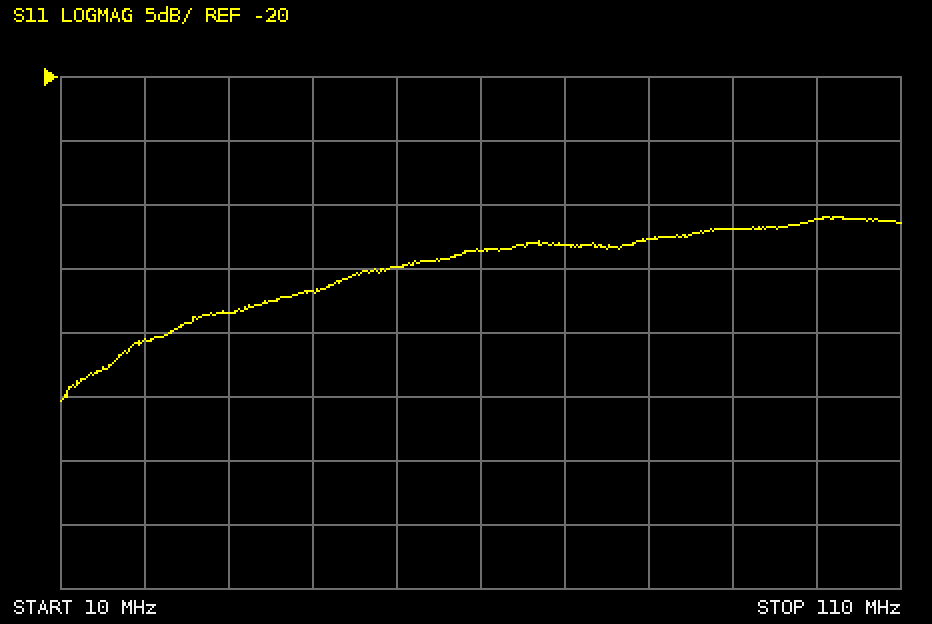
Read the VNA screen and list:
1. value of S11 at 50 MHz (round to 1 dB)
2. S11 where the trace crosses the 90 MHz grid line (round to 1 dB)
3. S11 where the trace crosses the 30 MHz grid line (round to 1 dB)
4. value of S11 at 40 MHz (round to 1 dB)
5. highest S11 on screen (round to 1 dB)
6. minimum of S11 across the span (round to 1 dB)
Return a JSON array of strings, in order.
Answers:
["-35 dB", "-32 dB", "-38 dB", "-37 dB", "-31 dB", "-45 dB"]
